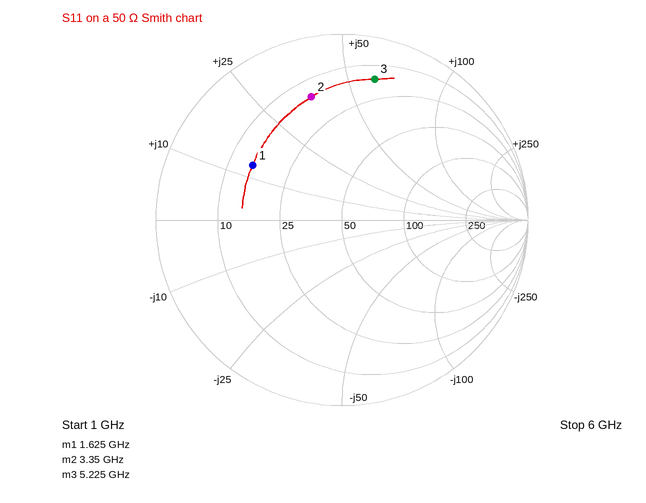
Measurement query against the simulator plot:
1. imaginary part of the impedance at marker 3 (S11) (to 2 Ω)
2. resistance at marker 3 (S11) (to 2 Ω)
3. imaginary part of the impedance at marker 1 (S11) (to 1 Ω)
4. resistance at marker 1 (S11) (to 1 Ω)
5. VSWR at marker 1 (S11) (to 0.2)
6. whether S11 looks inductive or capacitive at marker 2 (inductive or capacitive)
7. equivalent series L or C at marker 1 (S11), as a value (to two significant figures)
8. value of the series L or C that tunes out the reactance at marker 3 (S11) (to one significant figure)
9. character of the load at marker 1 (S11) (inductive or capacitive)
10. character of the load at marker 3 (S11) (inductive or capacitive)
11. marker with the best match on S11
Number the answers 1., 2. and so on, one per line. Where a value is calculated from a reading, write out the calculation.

1. +60 Ω
2. 16 Ω
3. +13 Ω
4. 15 Ω
5. 3.6
6. inductive
7. L = 13 Ω/(2π × 1.625 GHz) ≈ 1.3 nH
8. C = 1/(2π × 5.225 GHz × 60 Ω) ≈ 508 fF, so 500 fF to one significant figure
9. inductive
10. inductive
11. marker 1
